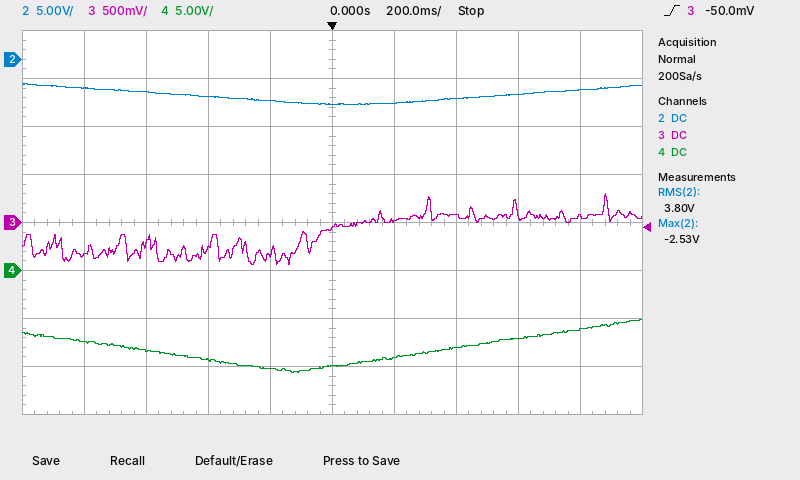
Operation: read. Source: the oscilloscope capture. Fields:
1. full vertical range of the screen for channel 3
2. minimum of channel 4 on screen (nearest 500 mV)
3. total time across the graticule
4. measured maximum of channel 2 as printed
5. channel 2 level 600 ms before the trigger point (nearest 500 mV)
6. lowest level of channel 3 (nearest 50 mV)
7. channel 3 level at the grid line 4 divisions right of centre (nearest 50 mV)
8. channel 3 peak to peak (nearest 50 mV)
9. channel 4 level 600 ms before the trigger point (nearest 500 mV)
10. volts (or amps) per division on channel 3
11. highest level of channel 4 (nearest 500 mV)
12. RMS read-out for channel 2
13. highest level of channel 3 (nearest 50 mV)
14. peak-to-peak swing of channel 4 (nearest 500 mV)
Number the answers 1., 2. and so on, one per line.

1. 4 V
2. -10.5 V
3. 2 s
4. -2.53 V
5. -3.5 V
6. -450 mV
7. 50 mV
8. 750 mV
9. -8.5 V
10. 500 mV
11. -5.0 V
12. 3.80 V
13. 300 mV
14. 5.5 V
